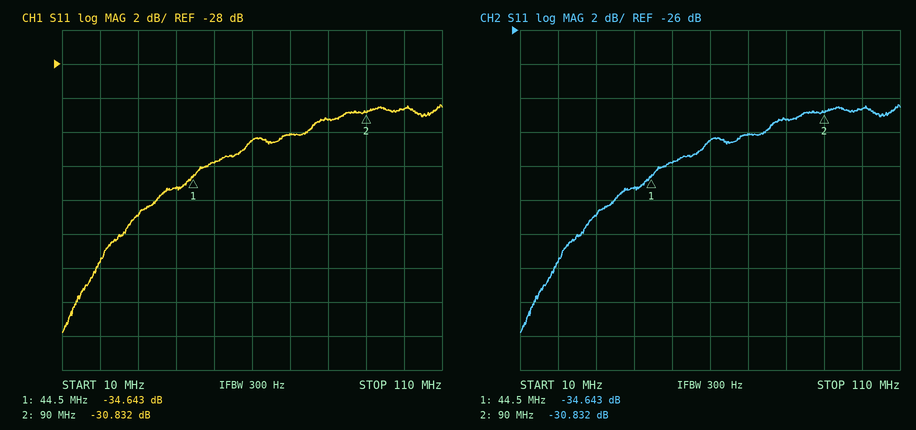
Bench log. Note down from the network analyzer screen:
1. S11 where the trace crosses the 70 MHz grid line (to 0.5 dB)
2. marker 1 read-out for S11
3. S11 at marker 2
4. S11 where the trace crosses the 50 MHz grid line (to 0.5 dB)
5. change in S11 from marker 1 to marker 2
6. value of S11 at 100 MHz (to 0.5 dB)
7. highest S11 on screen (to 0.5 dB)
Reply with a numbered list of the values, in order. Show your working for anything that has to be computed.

1. -32.0 dB
2. -34.643 dB
3. -30.832 dB
4. -34.0 dB
5. -30.832 − (-34.643) = 3.811 dB
6. -30.5 dB
7. -30.5 dB
